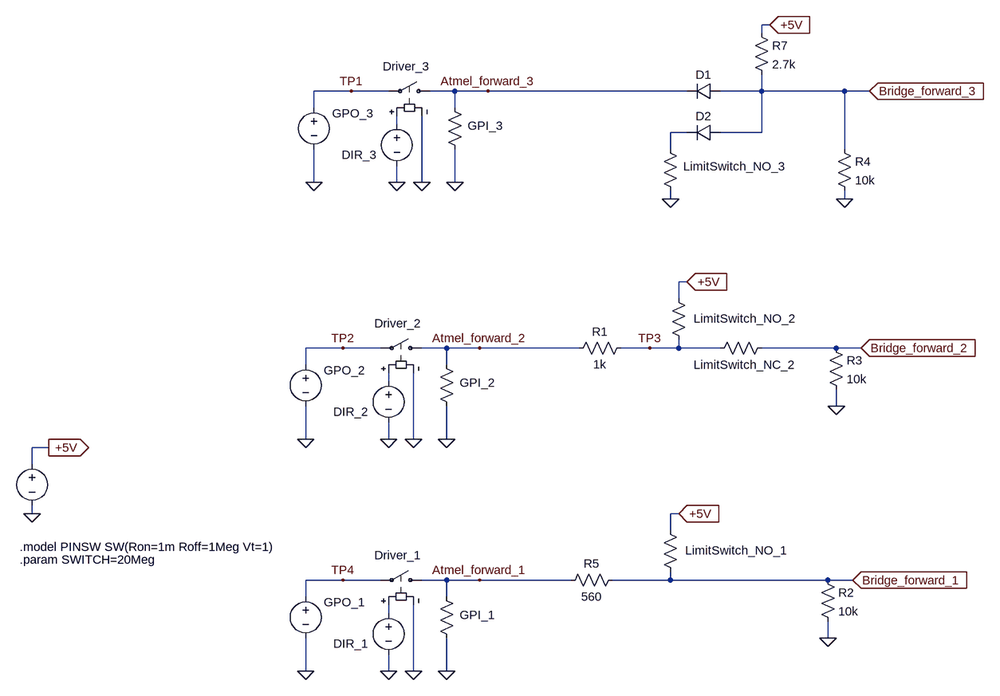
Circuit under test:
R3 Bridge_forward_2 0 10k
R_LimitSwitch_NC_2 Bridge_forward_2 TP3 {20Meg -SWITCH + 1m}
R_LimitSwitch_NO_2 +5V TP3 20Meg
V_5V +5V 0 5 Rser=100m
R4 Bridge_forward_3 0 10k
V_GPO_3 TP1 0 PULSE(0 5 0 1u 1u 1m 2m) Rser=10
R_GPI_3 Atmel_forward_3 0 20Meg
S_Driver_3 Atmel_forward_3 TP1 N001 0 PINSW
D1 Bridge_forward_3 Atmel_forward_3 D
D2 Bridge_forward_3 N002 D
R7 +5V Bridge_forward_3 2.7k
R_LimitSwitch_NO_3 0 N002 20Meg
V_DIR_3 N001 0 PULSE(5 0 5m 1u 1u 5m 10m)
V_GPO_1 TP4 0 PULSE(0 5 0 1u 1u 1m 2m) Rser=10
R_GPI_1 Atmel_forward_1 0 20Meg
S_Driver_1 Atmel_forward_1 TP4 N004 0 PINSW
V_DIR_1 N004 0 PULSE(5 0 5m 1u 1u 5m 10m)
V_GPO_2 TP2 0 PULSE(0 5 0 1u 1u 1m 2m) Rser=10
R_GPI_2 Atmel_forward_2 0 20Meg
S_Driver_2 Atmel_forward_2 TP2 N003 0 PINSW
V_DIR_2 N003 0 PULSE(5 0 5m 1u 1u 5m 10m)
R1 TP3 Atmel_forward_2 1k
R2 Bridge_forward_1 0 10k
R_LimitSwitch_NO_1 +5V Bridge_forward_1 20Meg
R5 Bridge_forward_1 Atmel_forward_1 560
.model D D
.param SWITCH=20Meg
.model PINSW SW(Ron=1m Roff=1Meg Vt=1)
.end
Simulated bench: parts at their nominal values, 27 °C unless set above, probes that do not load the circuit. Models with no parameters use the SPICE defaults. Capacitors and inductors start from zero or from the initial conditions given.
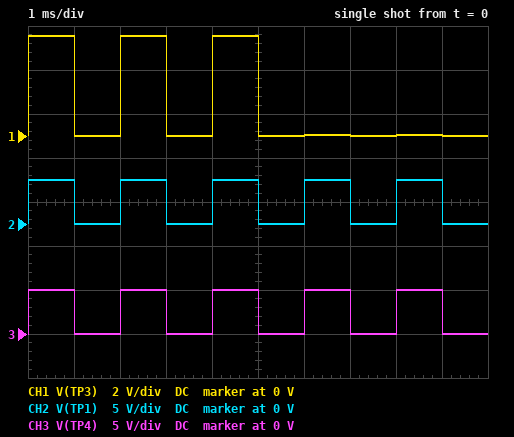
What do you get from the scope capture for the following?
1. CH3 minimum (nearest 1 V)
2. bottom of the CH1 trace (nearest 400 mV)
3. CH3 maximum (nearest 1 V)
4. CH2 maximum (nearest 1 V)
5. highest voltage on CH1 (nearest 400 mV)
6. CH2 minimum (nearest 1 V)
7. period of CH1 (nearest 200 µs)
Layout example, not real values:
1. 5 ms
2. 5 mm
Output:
1. 0 V
2. 0 V
3. 5 V
4. 5 V
5. 4.4 V
6. 0 V
7. 2.0 ms
